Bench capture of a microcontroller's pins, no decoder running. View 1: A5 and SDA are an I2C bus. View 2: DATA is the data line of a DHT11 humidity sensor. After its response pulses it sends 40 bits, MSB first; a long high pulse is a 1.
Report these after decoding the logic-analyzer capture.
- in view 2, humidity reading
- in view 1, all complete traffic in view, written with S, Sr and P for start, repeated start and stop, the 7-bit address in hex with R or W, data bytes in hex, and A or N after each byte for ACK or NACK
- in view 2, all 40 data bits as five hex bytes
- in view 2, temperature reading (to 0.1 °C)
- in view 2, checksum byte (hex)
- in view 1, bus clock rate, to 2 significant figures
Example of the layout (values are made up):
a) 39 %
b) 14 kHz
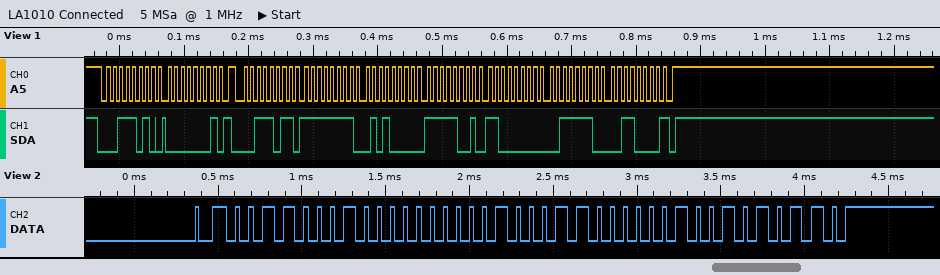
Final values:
a) 49 %
b) S 1DW A 01 A Sr 1DR A FF A 50 A F9 A C0 A 3E A 30 N P
c) 31 00 23 02 56
d) 35.2 °C
e) 0x56
f) 100 kHz
